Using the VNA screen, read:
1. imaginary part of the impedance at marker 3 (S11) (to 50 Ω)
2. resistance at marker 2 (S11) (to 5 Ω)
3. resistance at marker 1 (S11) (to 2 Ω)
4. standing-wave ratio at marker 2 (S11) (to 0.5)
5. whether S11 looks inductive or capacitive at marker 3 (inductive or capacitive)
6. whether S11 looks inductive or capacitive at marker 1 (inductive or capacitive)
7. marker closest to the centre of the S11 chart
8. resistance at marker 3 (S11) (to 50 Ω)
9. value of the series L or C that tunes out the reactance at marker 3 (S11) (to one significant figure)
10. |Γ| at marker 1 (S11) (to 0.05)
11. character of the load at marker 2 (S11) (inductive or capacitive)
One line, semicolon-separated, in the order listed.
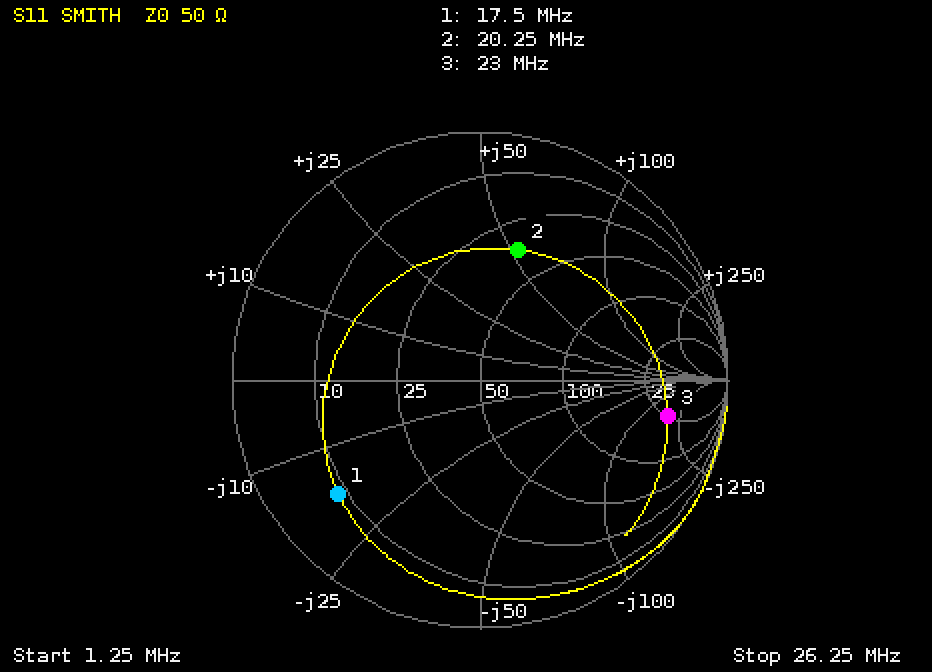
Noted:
-200 Ω; 35 Ω; 8 Ω; 3.5; capacitive; capacitive; marker 2; 250 Ω; 1 µH; 0.75; inductive
